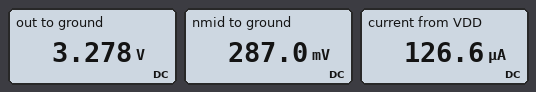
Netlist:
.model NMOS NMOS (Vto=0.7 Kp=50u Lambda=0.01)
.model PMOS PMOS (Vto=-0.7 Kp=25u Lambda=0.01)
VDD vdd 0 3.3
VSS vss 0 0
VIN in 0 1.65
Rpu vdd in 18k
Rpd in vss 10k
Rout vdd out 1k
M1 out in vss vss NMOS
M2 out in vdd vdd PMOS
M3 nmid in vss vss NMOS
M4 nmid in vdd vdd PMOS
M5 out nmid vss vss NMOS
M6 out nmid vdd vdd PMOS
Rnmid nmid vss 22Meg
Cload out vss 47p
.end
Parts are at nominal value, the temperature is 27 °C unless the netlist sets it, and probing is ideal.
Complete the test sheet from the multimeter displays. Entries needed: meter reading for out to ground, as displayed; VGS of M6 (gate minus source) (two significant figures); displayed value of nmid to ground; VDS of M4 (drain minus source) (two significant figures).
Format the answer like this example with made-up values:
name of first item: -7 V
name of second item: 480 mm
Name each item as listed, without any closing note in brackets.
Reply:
meter reading for out to ground, as displayed: 3.278 V
VGS of M6 (gate minus source): -3.0 V
displayed value of nmid to ground: 287.0 mV
VDS of M4 (drain minus source): -3.0 V
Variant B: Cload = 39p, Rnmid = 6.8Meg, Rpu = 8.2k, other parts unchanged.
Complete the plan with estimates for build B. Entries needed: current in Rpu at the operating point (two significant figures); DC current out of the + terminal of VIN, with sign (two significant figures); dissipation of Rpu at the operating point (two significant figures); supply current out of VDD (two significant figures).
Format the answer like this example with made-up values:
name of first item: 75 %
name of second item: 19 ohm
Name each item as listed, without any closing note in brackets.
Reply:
current in Rpu at the operating point: 200 µA
DC current out of the + terminal of VIN, with sign: -36 µA
dissipation of Rpu at the operating point: 330 µW
supply current out of VDD: 240 µA
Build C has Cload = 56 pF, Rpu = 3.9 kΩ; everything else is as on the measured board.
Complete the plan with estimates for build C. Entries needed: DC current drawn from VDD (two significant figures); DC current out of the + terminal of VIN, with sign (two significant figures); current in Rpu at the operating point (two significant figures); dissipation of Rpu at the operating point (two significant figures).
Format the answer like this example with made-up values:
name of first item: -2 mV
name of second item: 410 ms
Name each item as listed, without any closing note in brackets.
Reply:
DC current drawn from VDD: 460 µA
DC current out of the + terminal of VIN, with sign: -260 µA
current in Rpu at the operating point: 420 µA
dissipation of Rpu at the operating point: 700 µW
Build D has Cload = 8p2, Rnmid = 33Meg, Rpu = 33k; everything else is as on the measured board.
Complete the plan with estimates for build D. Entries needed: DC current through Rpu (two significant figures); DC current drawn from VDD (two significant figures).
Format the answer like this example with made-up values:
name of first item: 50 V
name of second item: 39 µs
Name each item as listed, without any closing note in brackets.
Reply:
DC current through Rpu: 50 µA
DC current drawn from VDD: 85 µA
